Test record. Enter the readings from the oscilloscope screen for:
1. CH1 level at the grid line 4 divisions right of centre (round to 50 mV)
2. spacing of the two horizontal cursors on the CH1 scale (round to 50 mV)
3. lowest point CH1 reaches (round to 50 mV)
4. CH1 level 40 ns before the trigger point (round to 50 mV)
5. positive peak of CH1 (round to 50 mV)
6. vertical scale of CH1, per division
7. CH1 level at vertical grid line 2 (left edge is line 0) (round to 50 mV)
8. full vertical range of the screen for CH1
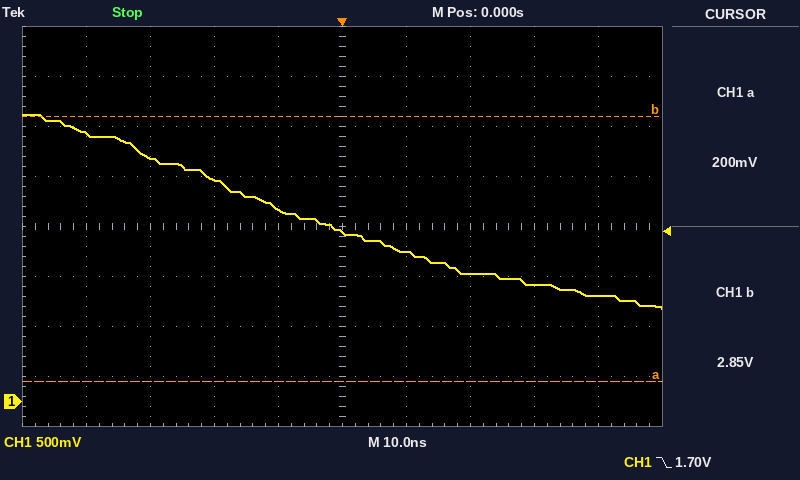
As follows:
1.05 V
2.65 V
950 mV
2.70 V
2.85 V
500 mV
2.45 V
4 V
